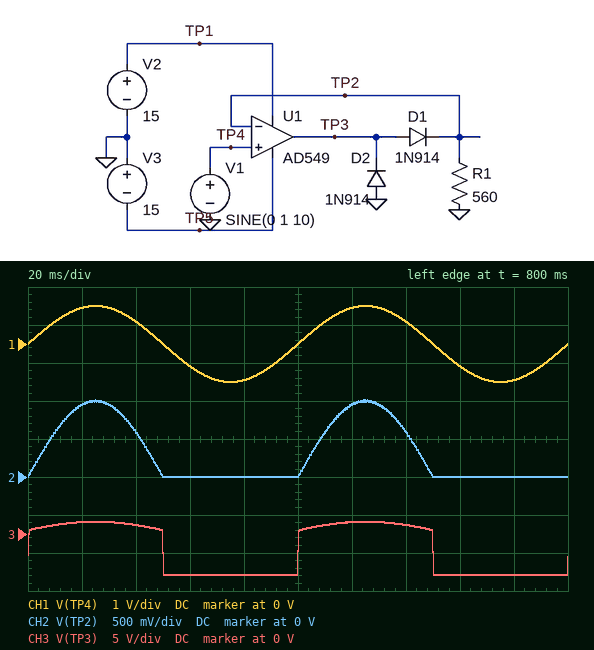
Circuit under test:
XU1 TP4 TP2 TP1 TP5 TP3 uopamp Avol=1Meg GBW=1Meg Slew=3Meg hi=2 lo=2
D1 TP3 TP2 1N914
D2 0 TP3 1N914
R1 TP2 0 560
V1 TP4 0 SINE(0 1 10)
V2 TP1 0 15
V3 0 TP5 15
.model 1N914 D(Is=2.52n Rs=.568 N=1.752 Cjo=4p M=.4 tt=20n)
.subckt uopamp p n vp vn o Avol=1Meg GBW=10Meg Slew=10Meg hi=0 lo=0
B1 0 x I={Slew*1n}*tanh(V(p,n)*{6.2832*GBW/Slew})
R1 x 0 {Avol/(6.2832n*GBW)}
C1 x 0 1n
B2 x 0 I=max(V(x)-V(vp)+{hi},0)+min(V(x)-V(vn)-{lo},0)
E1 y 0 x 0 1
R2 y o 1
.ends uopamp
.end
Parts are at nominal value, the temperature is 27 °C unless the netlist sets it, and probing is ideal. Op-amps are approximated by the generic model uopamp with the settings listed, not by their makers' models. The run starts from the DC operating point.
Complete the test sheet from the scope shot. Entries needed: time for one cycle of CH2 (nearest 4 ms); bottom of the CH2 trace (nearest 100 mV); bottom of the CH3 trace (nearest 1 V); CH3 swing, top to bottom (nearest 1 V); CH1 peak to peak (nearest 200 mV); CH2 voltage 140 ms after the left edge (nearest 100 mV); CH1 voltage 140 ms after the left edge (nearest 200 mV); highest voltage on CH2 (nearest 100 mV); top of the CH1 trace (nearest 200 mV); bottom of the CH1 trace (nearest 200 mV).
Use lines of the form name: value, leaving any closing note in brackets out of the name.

time for one cycle of CH2: 100 ms
bottom of the CH2 trace: 0 V
bottom of the CH3 trace: -5 V
CH3 swing, top to bottom: 7 V
CH1 peak to peak: 2.0 V
CH2 voltage 140 ms after the left edge: 600 mV
CH1 voltage 140 ms after the left edge: 600 mV
highest voltage on CH2: 1.0 V
top of the CH1 trace: 1.0 V
bottom of the CH1 trace: -1.0 V
